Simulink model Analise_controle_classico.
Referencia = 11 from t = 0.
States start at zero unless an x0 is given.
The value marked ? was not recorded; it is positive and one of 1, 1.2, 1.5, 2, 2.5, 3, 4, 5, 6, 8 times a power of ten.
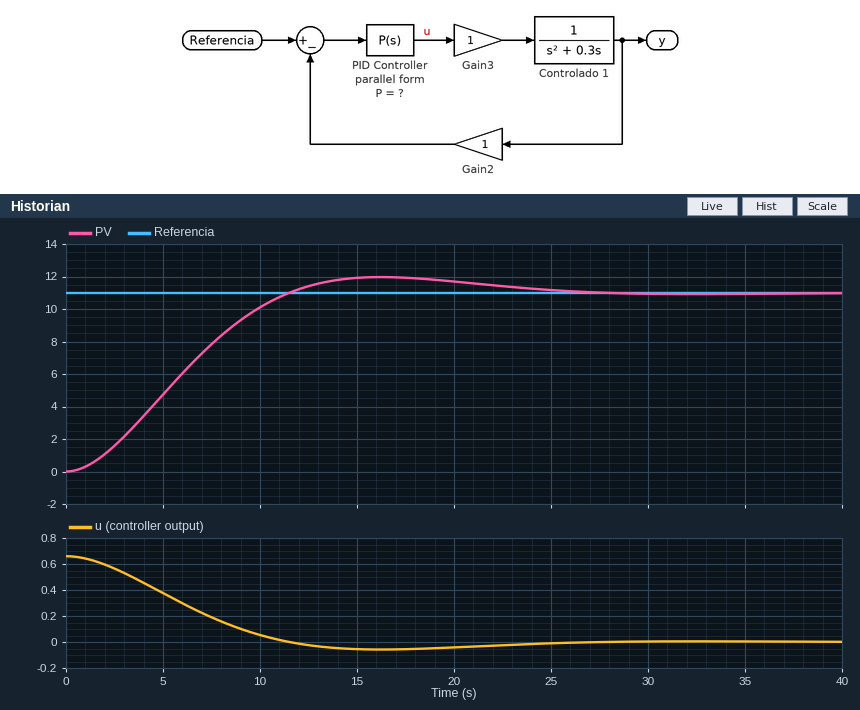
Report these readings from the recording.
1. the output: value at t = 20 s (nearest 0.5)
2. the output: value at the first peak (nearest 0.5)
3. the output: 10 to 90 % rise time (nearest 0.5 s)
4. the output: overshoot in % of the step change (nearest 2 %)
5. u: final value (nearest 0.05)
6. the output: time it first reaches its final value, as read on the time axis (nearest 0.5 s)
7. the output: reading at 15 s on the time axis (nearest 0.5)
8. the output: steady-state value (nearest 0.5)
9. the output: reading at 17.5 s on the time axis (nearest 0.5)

11.5
12.0
7.5 s
8 %
0.00
11.5 s
12.0
11.0
12.0
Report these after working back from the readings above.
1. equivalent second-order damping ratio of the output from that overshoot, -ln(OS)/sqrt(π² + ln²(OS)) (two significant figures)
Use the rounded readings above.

0.63
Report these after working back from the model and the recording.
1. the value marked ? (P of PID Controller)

0.06
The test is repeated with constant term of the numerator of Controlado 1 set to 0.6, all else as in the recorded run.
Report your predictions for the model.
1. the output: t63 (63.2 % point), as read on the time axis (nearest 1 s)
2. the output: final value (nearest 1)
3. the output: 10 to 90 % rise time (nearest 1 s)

10 s
11
13 s
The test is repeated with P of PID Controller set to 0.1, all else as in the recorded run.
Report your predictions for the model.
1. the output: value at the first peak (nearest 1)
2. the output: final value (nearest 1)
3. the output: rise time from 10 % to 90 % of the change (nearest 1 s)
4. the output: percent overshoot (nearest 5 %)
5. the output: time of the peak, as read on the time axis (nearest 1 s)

13
11
5 s
20 %
11 s
